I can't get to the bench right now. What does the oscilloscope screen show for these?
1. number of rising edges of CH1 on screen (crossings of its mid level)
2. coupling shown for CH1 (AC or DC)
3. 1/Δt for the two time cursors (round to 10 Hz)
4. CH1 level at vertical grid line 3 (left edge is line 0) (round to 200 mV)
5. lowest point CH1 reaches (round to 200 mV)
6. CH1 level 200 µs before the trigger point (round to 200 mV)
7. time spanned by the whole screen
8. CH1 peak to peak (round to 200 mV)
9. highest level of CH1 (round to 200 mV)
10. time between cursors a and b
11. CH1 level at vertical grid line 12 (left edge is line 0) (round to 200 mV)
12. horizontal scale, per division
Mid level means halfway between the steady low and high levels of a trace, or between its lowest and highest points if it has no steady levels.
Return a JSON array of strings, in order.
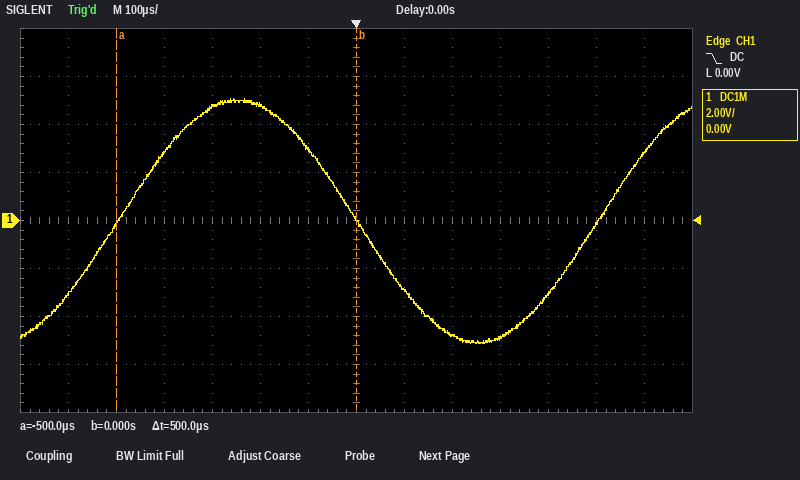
["2", "DC", "2.00 kHz", "2.8 V", "-5.2 V", "4.8 V", "1.4 ms", "10.2 V", "5.0 V", "500 µs", "-200 mV", "100 µs"]
